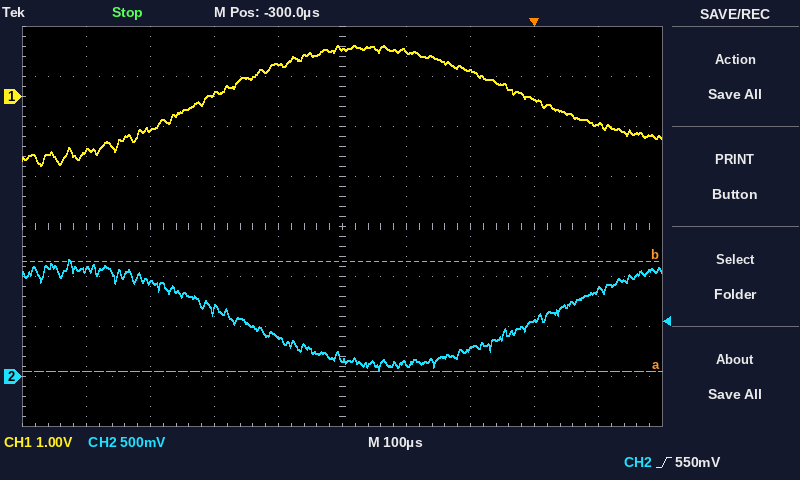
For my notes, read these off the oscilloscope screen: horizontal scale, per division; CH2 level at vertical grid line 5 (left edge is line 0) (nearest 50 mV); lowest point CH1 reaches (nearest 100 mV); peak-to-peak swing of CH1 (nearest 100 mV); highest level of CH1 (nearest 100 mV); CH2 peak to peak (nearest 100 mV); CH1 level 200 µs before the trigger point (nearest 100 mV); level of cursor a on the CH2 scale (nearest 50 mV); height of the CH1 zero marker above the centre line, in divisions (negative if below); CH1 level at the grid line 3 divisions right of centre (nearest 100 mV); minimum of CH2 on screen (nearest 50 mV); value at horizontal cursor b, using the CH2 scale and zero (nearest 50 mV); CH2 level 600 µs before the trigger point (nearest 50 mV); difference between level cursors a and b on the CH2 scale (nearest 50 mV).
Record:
100 µs
200 mV
-1.4 V
2.4 V
1.0 V
1.10 V
900 mV
50 mV
+2.6 div
-100 mV
50 mV
1.15 V
950 mV
1.10 V
